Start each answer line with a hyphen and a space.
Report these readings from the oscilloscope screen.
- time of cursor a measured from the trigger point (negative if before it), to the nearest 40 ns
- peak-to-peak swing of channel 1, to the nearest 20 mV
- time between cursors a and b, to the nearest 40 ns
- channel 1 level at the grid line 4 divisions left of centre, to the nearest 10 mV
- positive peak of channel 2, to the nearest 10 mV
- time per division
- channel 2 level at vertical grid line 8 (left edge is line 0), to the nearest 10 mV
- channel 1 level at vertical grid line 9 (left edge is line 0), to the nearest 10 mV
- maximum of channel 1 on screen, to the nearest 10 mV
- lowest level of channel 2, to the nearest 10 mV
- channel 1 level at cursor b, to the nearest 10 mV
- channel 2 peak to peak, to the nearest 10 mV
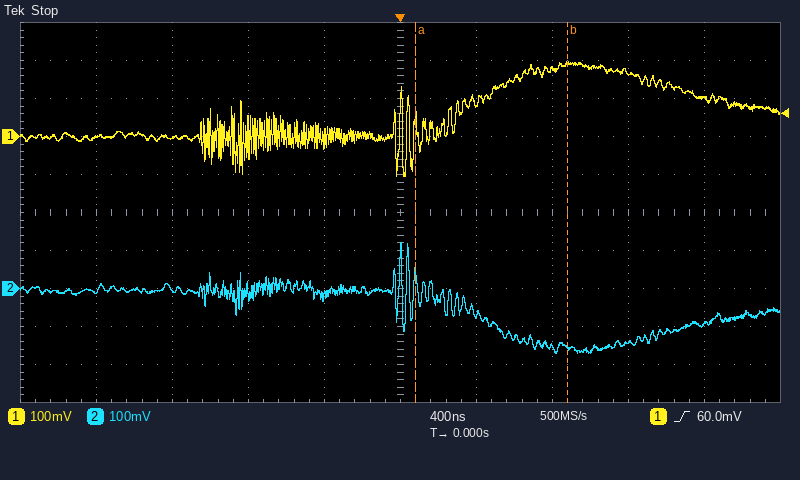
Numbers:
- +80 ns
- 300 mV
- 800 ns
- 0 mV
- 120 mV
- 400 ns
- -140 mV
- 100 mV
- 200 mV
- -170 mV
- 190 mV
- 290 mV
